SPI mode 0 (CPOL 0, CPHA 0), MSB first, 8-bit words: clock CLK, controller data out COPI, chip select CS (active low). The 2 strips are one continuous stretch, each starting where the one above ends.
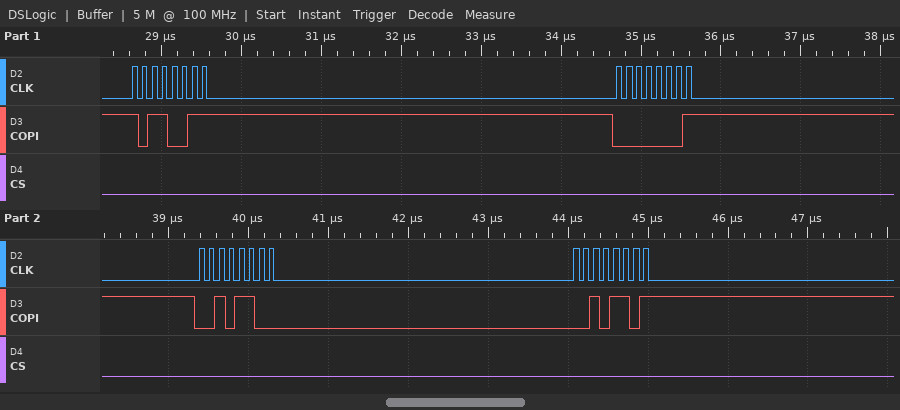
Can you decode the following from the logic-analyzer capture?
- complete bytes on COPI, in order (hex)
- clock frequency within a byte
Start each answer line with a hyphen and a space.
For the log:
- B3 01 2C 2D
- 8 MHz
